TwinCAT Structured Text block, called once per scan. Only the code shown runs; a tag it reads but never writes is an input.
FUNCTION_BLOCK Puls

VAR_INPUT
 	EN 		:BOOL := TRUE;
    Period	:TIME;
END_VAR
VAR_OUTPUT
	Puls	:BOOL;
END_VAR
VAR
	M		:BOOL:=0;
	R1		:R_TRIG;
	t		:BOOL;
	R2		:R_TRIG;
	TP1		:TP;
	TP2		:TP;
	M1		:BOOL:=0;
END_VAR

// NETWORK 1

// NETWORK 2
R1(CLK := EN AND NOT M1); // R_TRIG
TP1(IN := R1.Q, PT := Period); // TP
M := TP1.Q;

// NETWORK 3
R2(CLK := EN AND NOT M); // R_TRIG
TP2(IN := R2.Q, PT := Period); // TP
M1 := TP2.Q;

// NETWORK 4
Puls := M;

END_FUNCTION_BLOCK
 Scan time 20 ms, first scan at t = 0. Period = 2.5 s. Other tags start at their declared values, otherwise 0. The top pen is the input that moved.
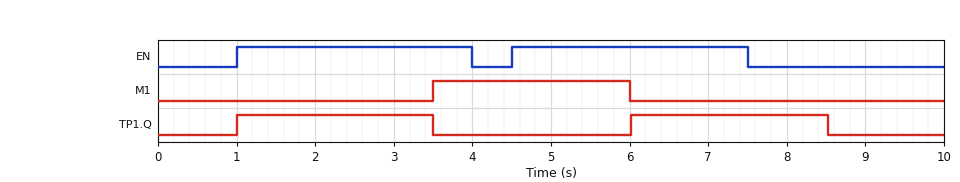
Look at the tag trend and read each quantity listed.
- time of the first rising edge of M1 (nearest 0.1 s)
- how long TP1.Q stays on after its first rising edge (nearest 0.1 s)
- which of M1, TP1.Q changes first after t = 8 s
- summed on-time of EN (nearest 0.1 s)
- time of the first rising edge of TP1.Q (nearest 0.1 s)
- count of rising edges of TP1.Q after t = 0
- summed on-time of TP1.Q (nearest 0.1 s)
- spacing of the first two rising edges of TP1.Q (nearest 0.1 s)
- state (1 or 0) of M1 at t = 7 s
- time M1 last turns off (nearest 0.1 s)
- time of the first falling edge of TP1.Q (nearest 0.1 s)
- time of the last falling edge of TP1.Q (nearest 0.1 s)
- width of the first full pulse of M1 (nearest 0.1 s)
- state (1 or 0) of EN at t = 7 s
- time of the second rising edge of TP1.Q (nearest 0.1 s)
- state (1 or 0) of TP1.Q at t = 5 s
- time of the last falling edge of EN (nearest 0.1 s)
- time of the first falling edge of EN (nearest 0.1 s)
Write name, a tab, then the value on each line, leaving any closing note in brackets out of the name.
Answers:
time of the first rising edge of M1	3.5 s
how long TP1.Q stays on after its first rising edge	2.5 s
which of M1, TP1.Q changes first after t = 8 s	TP1.Q
summed on-time of EN	6.0 s
time of the first rising edge of TP1.Q	1.0 s
count of rising edges of TP1.Q after t = 0	2
summed on-time of TP1.Q	5.0 s
spacing of the first two rising edges of TP1.Q	5.0 s
state (1 or 0) of M1 at t = 7 s	0
time M1 last turns off	6.0 s
time of the first falling edge of TP1.Q	3.5 s
time of the last falling edge of TP1.Q	8.5 s
width of the first full pulse of M1	2.5 s
state (1 or 0) of EN at t = 7 s	1
time of the second rising edge of TP1.Q	6.0 s
state (1 or 0) of TP1.Q at t = 5 s	0
time of the last falling edge of EN	7.5 s
time of the first falling edge of EN	4.0 s
